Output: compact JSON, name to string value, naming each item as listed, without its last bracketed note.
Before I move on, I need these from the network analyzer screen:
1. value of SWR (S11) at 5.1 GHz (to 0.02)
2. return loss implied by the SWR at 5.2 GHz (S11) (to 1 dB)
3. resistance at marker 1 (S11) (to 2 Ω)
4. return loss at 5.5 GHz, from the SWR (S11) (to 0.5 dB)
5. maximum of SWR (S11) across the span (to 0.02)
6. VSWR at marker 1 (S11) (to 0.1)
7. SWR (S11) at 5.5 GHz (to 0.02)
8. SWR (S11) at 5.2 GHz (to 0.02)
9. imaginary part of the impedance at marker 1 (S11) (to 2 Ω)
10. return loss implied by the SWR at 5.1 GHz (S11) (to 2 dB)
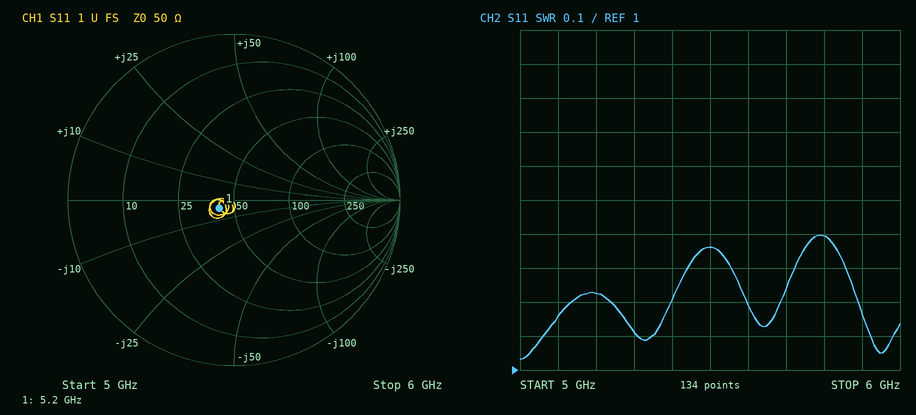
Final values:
{"value of SWR (S11) at 5.1 GHz": "1.16", "return loss implied by the SWR at 5.2 GHz (S11)": "20 dB", "resistance at marker 1 (S11)": "42 Ω", "return loss at 5.5 GHz, from the SWR (S11)": "16.5 dB", "maximum of SWR (S11) across the span": "1.40", "VSWR at marker 1 (S11)": "1.2", "SWR (S11) at 5.5 GHz": "1.36", "SWR (S11) at 5.2 GHz": "1.22", "imaginary part of the impedance at marker 1 (S11)": "-4 Ω", "return loss implied by the SWR at 5.1 GHz (S11)": "22 dB"}
